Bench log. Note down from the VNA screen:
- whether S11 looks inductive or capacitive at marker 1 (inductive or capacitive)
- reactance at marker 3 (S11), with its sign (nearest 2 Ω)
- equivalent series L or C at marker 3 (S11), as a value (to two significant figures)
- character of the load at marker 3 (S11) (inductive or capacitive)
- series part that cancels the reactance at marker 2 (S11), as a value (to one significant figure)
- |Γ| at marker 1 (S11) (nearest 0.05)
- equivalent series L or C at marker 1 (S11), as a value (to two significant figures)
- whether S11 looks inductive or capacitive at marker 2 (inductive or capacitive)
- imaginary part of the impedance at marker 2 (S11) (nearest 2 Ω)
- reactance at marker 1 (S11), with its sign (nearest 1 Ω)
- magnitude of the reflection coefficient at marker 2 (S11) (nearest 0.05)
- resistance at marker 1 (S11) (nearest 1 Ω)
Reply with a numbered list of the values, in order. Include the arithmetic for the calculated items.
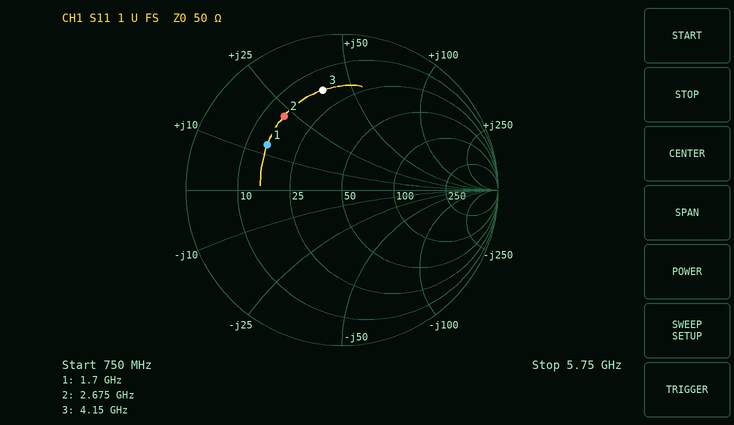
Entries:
1. inductive
2. +38 Ω
3. L = 38 Ω/(2π × 4.15 GHz) ≈ 1.5 nH
4. inductive
5. C = 1/(2π × 2.675 GHz × 22 Ω) ≈ 3 pF
6. 0.55
7. L = 13 Ω/(2π × 1.7 GHz) ≈ 1.2 nH
8. inductive
9. +22 Ω
10. +13 Ω
11. 0.60
12. 15 Ω
